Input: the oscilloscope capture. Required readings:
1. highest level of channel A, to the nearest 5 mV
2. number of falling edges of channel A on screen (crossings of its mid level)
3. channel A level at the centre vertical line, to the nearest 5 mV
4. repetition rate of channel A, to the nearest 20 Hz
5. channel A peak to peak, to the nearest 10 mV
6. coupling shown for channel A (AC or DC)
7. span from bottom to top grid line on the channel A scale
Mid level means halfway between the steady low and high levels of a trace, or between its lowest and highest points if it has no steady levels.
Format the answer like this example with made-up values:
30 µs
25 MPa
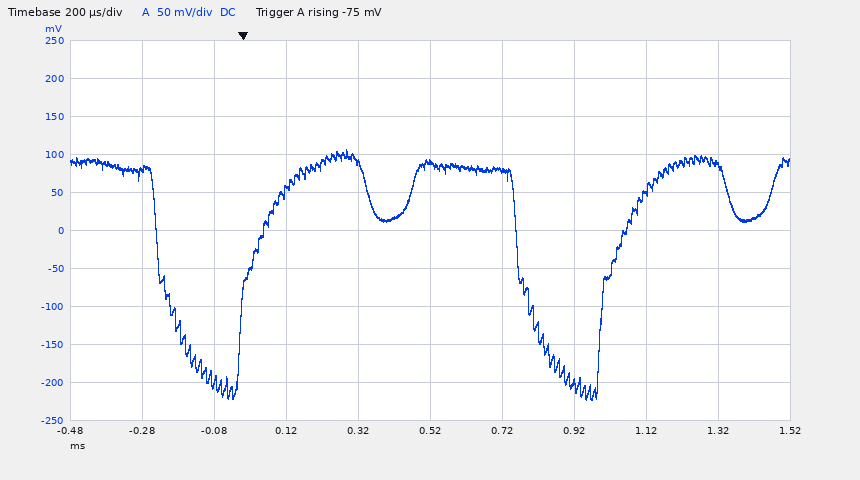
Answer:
105 mV
2
90 mV
1.00 kHz
330 mV
DC
500 mV
